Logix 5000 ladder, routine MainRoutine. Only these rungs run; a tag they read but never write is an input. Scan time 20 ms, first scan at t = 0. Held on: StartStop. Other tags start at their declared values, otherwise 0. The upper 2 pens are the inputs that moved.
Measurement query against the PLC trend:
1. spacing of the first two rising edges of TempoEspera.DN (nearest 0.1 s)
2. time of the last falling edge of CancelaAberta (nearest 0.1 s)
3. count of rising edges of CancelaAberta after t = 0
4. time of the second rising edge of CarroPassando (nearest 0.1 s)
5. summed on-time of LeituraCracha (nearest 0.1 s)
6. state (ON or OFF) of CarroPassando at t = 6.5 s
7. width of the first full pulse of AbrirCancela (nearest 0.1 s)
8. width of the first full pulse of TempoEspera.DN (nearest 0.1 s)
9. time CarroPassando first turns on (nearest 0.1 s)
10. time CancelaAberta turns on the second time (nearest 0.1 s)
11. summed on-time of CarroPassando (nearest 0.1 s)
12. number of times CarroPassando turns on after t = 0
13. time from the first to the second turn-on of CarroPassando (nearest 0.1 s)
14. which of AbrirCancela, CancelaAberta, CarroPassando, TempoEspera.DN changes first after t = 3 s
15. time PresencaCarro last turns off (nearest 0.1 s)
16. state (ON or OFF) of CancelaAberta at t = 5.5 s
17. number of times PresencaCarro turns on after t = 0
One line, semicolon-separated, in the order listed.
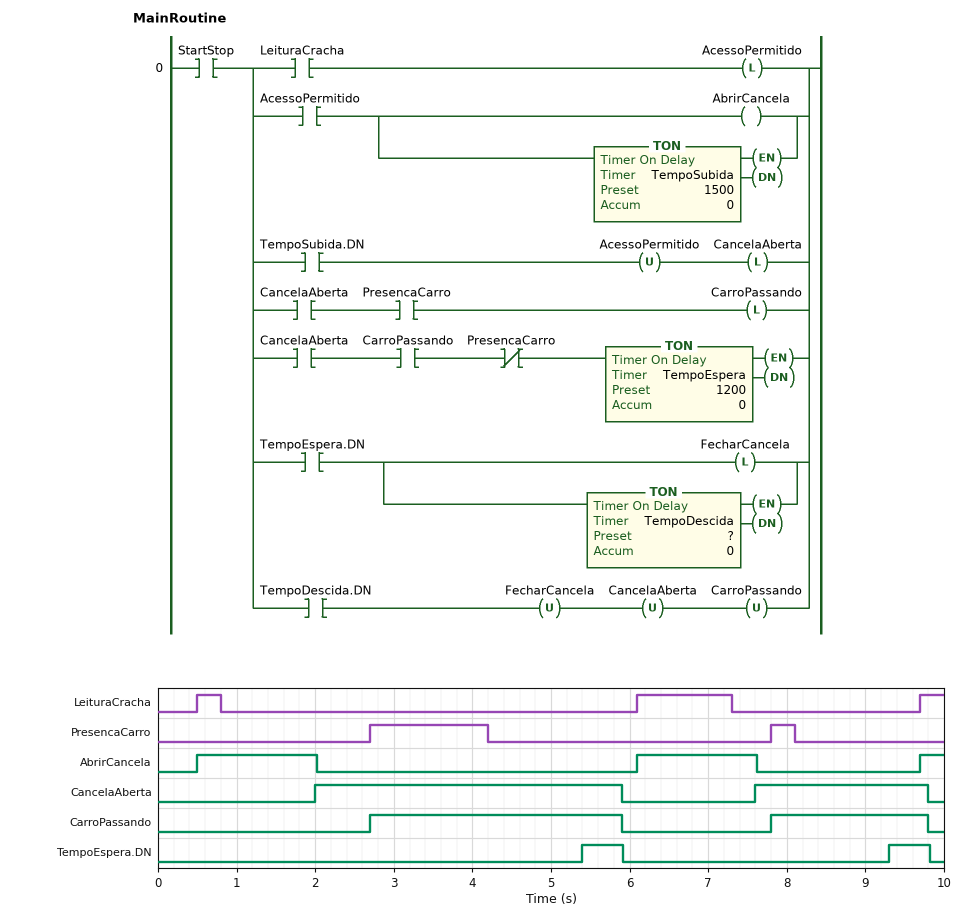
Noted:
3.9 s; 9.8 s; 2; 7.8 s; 1.8 s; OFF; 1.5 s; 0.5 s; 2.7 s; 7.6 s; 5.2 s; 2; 5.1 s; TempoEspera.DN; 8.1 s; ON; 2
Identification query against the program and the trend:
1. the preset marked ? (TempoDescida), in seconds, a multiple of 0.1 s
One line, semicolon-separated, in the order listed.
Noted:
0.5 s
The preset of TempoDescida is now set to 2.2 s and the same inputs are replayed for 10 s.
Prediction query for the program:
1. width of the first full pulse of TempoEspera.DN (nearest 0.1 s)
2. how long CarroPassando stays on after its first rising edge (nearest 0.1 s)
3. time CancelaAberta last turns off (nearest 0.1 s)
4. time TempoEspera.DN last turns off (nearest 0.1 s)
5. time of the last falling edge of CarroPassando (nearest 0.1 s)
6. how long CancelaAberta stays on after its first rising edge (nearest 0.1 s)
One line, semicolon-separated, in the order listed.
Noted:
2.2 s; 4.9 s; 7.6 s; 7.6 s; 7.6 s; 5.6 s
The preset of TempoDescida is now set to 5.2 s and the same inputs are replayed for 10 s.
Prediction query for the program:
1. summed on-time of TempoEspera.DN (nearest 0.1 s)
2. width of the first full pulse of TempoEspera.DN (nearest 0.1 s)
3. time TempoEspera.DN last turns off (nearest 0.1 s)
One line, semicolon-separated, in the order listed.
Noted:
3.1 s; 2.4 s; 7.8 s
